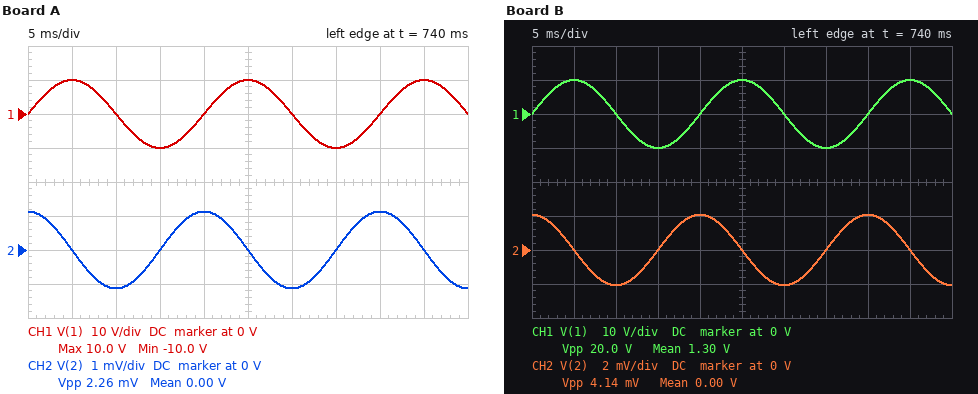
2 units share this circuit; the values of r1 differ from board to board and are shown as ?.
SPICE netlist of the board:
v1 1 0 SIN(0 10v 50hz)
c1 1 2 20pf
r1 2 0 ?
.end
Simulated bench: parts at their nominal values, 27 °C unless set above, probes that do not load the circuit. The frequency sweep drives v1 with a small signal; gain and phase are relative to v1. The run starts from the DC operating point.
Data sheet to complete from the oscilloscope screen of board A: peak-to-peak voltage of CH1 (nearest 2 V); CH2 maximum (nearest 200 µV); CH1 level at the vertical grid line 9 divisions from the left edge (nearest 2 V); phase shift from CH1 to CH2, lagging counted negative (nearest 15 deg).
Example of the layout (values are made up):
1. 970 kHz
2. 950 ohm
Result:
1. 20 V
2. 1.2 mV
3. 10 V
4. 90 deg
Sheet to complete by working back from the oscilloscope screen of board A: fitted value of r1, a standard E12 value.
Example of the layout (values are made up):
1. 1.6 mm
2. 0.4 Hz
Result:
1. 18 kΩ
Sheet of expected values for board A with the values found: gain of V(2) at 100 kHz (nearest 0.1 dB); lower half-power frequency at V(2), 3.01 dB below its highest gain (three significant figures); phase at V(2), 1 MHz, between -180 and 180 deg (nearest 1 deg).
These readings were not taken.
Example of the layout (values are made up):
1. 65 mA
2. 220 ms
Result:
1. -13.1 dB
2. 442 kHz
3. 24 deg
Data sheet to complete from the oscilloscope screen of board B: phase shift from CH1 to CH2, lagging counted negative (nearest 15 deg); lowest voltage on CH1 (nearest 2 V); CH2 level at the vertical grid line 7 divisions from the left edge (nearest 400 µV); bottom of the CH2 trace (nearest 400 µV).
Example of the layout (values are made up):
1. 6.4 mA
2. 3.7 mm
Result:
1. 90 deg
2. -10 V
3. 0 V
4. -2.0 mV
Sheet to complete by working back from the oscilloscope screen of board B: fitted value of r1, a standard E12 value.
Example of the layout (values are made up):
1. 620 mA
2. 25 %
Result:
1. 33 kΩ
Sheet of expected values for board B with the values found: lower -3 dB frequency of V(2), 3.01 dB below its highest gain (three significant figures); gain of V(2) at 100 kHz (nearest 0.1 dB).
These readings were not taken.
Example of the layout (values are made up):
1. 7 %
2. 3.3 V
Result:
1. 241 kHz
2. -8.3 dB
